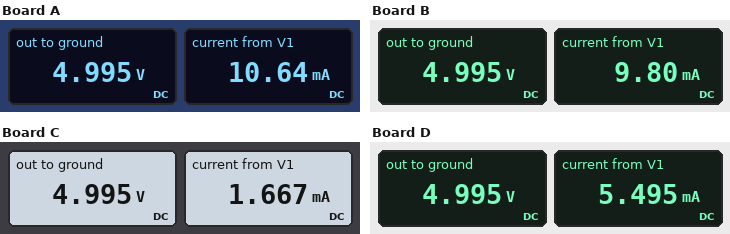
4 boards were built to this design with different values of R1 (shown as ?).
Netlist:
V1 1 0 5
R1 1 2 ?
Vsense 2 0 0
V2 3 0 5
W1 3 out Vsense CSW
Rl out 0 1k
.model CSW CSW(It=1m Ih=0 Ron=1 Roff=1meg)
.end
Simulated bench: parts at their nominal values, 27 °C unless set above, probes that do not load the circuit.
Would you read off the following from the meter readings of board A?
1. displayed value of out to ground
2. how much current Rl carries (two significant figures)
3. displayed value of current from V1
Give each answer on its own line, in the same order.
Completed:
4.995 V
5.0 mA
10.64 mA
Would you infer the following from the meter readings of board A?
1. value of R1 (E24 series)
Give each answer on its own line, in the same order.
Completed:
470 Ω
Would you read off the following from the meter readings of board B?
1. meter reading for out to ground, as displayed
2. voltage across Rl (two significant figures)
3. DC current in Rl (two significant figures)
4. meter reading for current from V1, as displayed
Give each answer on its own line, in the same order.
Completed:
4.995 V
5.0 V
5.0 mA
9.80 mA
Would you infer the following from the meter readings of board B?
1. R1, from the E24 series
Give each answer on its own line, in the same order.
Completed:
510 Ω
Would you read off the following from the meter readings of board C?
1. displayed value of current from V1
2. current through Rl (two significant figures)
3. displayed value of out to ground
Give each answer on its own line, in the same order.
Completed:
1.667 mA
5.0 mA
4.995 V
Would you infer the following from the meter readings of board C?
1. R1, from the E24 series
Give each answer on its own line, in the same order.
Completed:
3 kΩ
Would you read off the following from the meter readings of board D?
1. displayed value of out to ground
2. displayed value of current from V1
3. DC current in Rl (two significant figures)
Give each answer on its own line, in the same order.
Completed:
4.995 V
5.495 mA
5.0 mA
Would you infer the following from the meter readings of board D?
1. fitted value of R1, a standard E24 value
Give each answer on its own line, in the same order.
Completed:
910 Ω
